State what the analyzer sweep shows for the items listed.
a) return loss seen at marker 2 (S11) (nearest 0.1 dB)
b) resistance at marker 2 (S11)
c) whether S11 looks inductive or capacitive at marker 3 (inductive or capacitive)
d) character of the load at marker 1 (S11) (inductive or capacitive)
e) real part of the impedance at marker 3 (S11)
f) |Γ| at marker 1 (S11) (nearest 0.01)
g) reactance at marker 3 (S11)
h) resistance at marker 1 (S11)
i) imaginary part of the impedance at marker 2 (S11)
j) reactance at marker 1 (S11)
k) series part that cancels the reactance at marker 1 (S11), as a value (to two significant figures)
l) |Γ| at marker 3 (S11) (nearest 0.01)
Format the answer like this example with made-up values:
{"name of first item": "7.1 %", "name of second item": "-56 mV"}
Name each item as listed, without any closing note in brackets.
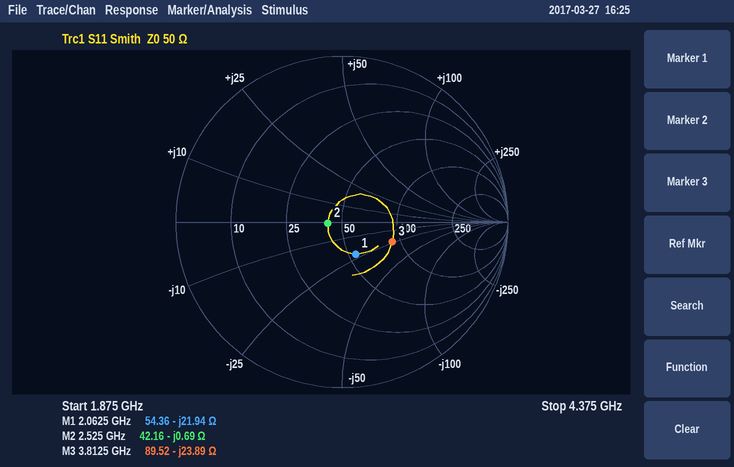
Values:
{"return loss seen at marker 2 (S11)": "21.4 dB", "resistance at marker 2": "42.16 Ω", "whether S11 looks inductive or capacitive at marker 3": "capacitive", "character of the load at marker 1 (S11)": "capacitive", "real part of the impedance at marker 3": "89.52 Ω", "|Γ| at marker 1 (S11)": "0.21", "reactance at marker 3": "-23.89 Ω", "resistance at marker 1": "54.36 Ω", "imaginary part of the impedance at marker 2": "-0.69 Ω", "reactance at marker 1": "-21.94 Ω", "series part that cancels the reactance at marker 1 (S11), as a value": "1.7 nH", "|Γ| at marker 3 (S11)": "0.33"}
